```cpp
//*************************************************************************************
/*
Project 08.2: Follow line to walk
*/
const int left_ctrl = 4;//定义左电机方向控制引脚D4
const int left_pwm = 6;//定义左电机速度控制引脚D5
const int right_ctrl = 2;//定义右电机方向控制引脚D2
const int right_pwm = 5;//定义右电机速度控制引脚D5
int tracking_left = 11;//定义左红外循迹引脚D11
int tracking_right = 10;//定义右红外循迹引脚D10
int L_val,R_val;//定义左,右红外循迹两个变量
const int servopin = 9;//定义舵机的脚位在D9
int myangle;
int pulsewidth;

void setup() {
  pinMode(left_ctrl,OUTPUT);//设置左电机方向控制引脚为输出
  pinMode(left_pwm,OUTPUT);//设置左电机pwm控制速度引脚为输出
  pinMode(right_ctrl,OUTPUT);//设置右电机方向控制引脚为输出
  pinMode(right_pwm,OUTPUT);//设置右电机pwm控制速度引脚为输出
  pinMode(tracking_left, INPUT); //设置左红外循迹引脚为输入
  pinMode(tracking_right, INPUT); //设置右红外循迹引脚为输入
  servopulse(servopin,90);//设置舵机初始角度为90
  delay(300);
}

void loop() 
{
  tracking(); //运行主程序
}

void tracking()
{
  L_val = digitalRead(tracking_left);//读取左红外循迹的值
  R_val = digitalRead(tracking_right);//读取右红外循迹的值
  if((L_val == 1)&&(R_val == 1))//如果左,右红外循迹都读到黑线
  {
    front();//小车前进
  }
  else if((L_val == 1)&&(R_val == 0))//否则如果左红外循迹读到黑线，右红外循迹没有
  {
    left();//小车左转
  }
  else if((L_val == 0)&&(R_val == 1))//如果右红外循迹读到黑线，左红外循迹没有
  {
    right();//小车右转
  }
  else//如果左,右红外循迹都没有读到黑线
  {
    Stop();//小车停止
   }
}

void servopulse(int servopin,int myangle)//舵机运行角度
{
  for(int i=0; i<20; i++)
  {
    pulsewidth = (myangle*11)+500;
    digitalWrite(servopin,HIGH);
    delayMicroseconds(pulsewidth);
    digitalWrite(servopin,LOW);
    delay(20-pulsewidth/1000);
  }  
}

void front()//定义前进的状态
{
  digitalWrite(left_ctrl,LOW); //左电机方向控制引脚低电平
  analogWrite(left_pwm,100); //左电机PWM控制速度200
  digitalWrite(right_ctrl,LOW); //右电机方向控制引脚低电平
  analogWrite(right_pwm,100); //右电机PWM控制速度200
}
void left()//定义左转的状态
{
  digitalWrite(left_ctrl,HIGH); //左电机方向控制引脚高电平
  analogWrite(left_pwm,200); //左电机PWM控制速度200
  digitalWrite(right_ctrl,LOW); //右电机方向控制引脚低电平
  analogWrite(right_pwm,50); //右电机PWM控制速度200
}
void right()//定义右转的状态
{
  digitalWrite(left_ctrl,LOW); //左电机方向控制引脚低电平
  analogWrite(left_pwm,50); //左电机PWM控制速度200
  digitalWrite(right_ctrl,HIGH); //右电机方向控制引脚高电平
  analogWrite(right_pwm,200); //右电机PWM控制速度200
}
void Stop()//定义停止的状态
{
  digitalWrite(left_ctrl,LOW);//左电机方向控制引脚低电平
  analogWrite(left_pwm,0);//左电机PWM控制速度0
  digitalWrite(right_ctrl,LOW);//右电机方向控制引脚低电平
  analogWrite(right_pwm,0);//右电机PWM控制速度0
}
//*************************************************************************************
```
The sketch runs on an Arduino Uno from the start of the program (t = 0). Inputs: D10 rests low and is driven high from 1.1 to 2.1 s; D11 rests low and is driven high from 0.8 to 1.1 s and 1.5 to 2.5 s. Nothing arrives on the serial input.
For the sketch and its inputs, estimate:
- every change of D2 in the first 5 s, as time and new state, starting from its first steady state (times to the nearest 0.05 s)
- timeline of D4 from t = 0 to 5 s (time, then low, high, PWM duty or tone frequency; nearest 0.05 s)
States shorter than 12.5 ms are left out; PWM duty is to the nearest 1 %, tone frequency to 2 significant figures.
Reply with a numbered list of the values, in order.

1. 0 s low; 1.1 s high; 1.5 s low
2. 0 s low; 0.8 s high; 1.1 s low; 2.1 s high; 2.5 s low
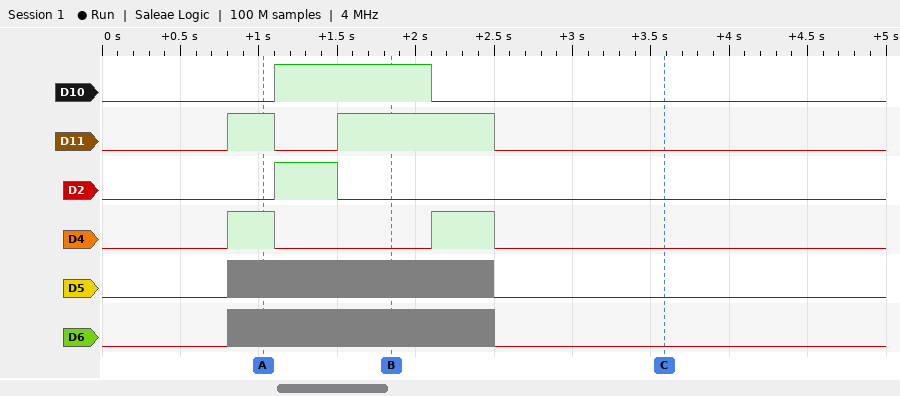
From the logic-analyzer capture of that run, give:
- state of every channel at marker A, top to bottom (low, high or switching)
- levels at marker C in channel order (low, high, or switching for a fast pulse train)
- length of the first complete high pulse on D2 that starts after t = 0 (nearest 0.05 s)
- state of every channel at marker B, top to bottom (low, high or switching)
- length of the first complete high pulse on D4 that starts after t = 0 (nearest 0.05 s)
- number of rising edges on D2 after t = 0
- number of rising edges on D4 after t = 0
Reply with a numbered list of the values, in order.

1. D10 low, D11 high, D2 low, D4 high, D5 switching, D6 switching
2. D10 low, D11 low, D2 low, D4 low, D5 low, D6 low
3. 0.40 s
4. D10 high, D11 high, D2 low, D4 low, D5 switching, D6 switching
5. 0.30 s
6. 1
7. 2
